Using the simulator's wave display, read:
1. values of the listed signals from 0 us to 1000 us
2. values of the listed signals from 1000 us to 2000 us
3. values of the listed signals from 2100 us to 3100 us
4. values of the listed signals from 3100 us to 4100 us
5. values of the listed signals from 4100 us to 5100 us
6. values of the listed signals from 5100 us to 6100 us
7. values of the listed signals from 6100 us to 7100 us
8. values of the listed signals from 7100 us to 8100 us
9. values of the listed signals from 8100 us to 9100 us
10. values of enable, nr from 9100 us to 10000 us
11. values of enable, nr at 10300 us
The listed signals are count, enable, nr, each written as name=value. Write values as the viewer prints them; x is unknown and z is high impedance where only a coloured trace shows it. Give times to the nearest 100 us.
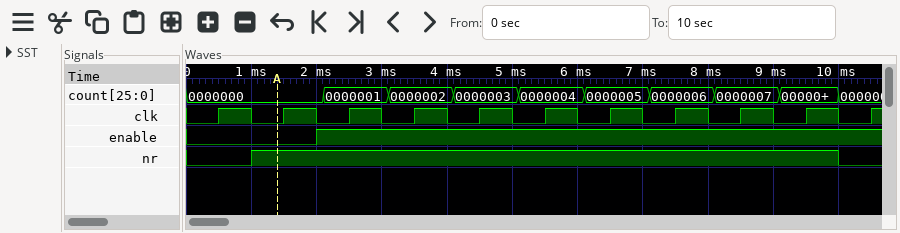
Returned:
count=0000000, enable=0, nr=0
count=0000000, enable=0, nr=1
count=0000001, enable=1, nr=1
count=0000002, enable=1, nr=1
count=0000003, enable=1, nr=1
count=0000004, enable=1, nr=1
count=0000005, enable=1, nr=1
count=0000006, enable=1, nr=1
count=0000007, enable=1, nr=1
enable=1, nr=1
enable=1, nr=0
